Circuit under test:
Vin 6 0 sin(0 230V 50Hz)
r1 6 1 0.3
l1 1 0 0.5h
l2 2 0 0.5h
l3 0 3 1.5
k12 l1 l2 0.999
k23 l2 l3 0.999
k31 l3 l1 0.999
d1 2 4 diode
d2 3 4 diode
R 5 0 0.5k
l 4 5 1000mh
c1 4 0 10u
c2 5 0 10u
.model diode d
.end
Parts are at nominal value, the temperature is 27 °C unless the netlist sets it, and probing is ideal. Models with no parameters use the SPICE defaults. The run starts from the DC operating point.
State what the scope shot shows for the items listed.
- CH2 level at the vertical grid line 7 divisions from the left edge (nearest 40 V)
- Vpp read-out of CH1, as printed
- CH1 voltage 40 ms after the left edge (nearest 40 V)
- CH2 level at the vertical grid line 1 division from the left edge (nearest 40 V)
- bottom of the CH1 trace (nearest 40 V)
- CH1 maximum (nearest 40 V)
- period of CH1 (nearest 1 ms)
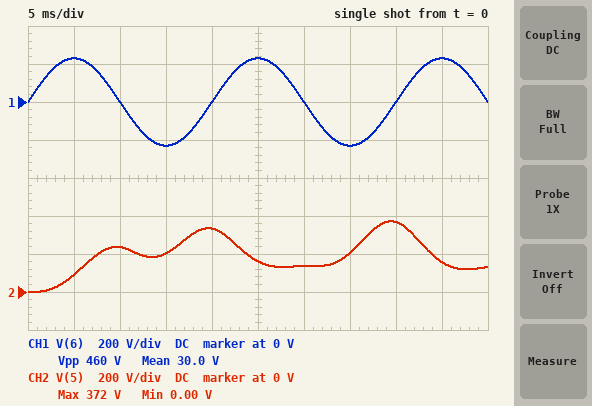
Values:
200 V
460 V
0 V
80 V
-240 V
240 V
20 ms
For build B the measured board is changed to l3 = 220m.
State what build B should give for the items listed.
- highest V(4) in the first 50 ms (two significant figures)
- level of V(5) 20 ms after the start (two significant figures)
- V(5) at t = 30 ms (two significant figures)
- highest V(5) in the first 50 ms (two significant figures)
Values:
230 V
89 V
210 V
240 V
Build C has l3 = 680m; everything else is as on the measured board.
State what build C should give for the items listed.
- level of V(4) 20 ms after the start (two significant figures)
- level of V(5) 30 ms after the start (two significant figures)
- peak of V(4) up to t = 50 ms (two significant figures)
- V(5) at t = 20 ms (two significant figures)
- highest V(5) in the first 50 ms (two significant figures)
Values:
75 V
170 V
270 V
200 V
240 V
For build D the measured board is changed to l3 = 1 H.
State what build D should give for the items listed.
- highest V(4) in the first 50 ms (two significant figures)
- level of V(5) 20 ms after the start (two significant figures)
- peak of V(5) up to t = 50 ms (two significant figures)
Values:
330 V
260 V
290 V
